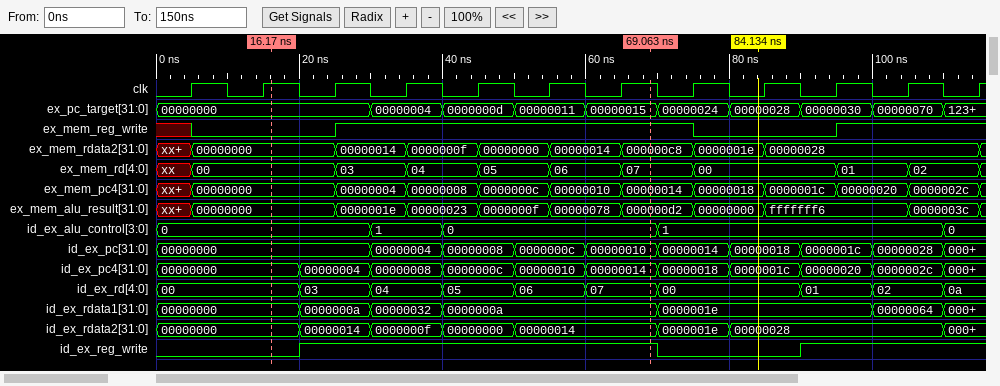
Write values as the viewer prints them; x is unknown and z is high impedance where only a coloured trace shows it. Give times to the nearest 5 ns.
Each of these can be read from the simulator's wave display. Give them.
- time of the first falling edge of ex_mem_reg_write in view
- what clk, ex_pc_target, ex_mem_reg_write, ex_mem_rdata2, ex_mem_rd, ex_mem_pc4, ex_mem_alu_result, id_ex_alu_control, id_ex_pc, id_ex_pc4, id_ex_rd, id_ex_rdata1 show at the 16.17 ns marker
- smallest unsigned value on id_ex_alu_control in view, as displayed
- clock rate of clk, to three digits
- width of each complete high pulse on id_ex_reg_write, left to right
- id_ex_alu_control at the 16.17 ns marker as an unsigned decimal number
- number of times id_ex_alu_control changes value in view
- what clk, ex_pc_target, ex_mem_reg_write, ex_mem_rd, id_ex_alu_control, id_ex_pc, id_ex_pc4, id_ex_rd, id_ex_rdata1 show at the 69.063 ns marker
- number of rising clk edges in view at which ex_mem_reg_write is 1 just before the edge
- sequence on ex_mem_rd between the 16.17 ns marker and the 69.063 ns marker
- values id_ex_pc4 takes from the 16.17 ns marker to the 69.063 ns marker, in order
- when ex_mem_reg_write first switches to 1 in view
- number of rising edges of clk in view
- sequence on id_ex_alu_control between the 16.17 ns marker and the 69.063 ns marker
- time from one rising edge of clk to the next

75 ns
clk=1, ex_pc_target=00000000, ex_mem_reg_write=0, ex_mem_rdata2=00000000, ex_mem_rd=00, ex_mem_pc4=00000000, ex_mem_alu_result=00000000, id_ex_alu_control=0, id_ex_pc=00000000, id_ex_pc4=00000000, id_ex_rd=00, id_ex_rdata1=00000000
0
100 MHz
50 ns
0
4
clk=1, ex_pc_target=00000015, ex_mem_reg_write=1, ex_mem_rd=07, id_ex_alu_control=0, id_ex_pc=00000010, id_ex_pc4=00000014, id_ex_rd=07, id_ex_rdata1=0000000a
7
00, 03, 04, 05, 06, 07
00000000, 00000004, 00000008, 0000000c, 00000010, 00000014
25 ns
12
0, 1, 0
10 ns
